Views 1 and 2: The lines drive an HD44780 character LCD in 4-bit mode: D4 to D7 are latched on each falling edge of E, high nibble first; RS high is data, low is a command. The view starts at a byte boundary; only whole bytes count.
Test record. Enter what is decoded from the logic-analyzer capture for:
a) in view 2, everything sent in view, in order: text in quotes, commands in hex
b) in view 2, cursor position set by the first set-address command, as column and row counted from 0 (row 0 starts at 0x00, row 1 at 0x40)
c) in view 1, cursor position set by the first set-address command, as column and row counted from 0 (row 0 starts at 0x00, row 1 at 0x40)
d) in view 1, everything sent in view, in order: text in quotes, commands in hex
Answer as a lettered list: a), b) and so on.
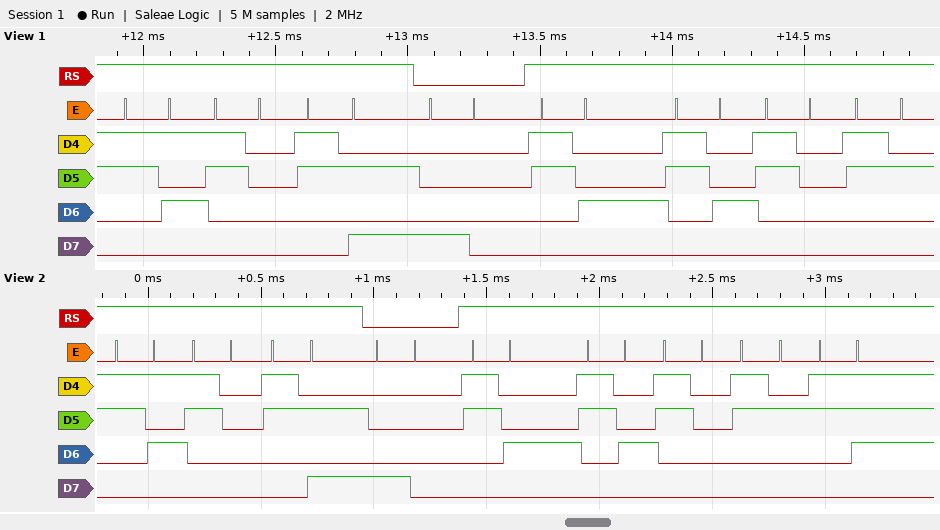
a) "50:" 0x80 "44027"
b) column 0, row 0
c) column 0, row 0
d) "50:" 0x80 "4402"
